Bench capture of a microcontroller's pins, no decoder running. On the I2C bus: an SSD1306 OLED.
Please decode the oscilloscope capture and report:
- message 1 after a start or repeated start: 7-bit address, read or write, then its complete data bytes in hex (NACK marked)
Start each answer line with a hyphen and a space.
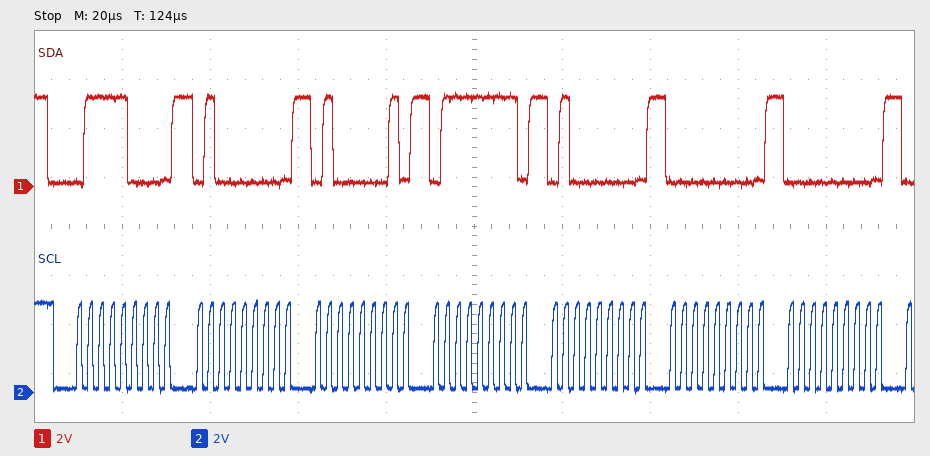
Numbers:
- 0x3C write: 40 41 7F 40 00 00
